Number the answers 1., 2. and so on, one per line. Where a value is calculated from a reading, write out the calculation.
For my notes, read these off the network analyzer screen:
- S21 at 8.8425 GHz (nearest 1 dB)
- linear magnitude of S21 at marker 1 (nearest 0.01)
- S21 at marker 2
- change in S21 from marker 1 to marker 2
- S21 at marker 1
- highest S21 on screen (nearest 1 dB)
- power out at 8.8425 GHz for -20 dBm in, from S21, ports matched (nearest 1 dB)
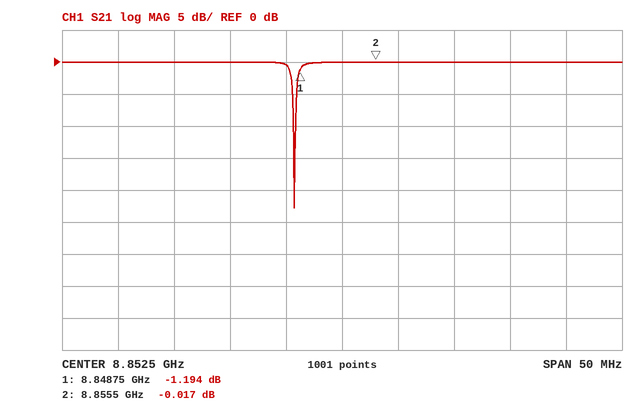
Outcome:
1. 0 dB
2. 10^(-1.194/20) ≈ 0.87
3. -0.017 dB
4. -0.017 − (-1.194) = 1.177 dB
5. -1.194 dB
6. 0 dB
7. -20 dBm + (0 dB) = -20 dBm
